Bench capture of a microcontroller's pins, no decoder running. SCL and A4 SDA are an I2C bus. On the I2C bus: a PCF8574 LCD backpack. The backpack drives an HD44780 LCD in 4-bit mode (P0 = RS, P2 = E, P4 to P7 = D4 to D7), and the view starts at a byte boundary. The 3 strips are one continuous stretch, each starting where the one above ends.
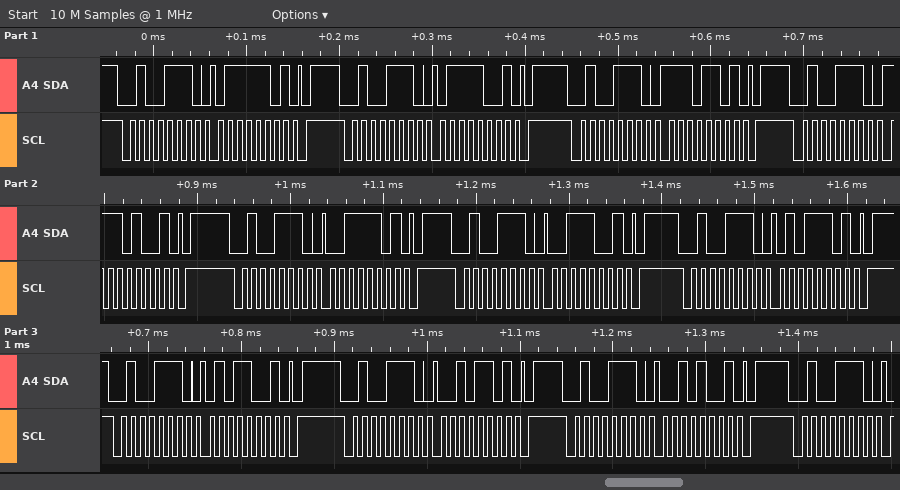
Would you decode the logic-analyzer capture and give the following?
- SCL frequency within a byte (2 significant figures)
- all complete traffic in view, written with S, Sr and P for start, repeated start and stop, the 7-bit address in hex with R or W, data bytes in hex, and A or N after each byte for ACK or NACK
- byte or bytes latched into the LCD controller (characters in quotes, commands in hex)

100 kHz
S 27W A 7D A P S 27W A 79 A P S 27W A ED A P S 27W A E9 A P S 27W A 3D A P S 27W A 39 A P S 27W A 5D A P S 27W A 59 A P S 27W A 2D A P S 27W A 29 A P S 27W A
data 0x7E '5'
